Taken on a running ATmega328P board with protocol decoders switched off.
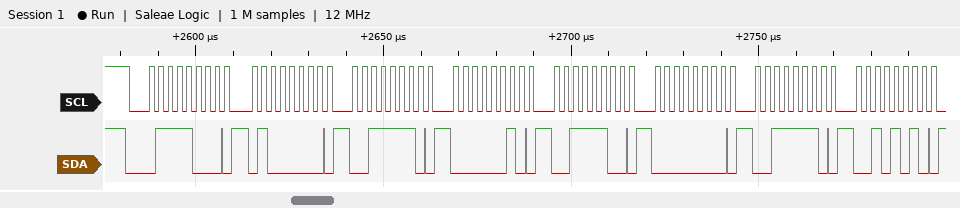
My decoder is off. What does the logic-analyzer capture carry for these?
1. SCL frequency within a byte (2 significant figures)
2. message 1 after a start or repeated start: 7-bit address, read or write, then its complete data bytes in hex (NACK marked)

400 kHz
0x3C write: 40 3E 02 3C 00 3E 2A
